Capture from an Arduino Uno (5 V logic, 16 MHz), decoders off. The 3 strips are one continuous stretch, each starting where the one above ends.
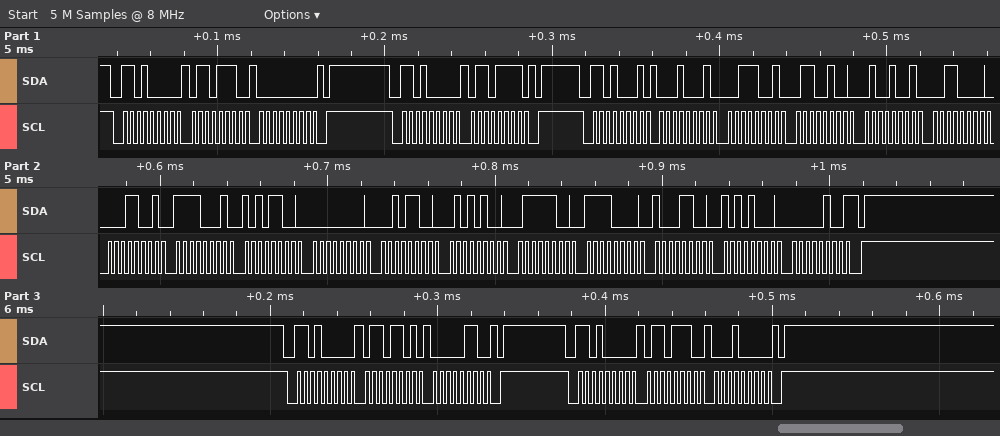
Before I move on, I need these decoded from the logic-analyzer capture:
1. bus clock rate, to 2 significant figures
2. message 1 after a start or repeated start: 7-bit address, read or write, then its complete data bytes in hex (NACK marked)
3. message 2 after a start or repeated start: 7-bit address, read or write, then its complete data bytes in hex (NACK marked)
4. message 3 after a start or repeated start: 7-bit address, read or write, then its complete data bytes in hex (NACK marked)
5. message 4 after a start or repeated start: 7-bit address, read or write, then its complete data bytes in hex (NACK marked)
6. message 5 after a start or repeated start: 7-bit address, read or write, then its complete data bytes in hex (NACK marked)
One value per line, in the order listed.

250 kHz
0x68 write: 6E 00
0x68 write: 6F
0x68 read: 11 39 64 49 30 19 F1 AC 00 2C 54 7C F0 8C A8 04 NACK
0x68 write: 6D 06
0x68 write: 6E 10
